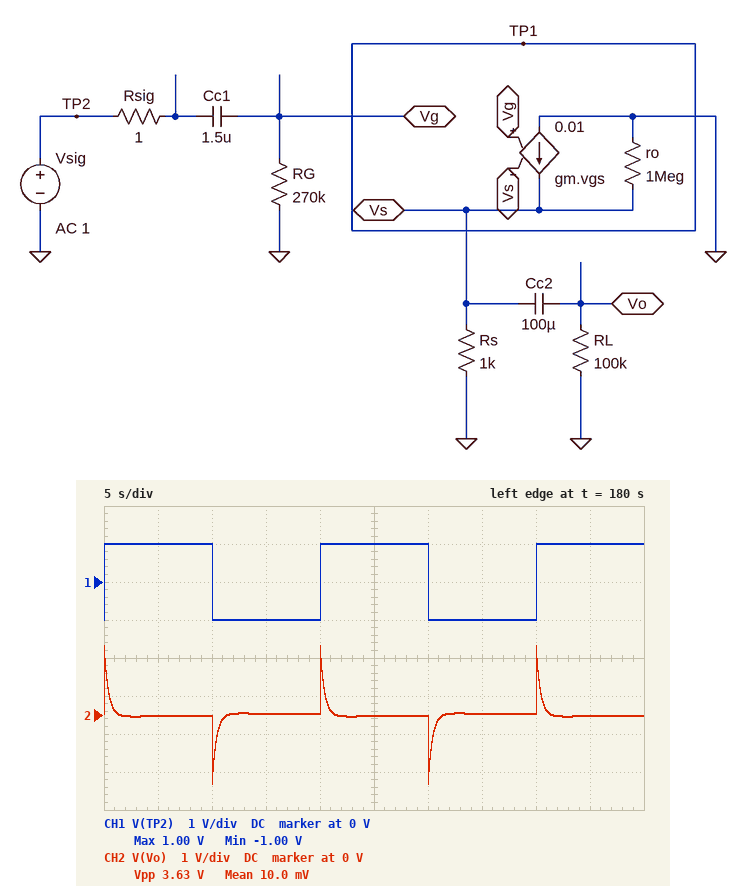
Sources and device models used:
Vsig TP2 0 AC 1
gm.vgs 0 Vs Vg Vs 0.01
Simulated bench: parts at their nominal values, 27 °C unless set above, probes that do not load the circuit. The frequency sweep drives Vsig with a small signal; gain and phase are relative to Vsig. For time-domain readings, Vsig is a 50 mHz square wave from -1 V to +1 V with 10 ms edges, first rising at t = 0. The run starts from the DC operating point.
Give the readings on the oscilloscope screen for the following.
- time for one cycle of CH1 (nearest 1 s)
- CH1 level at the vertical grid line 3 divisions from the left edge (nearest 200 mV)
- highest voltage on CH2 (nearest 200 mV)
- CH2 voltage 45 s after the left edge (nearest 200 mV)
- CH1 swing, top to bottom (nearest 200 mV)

20 s
-1.0 V
1.8 V
0 V
2.0 V
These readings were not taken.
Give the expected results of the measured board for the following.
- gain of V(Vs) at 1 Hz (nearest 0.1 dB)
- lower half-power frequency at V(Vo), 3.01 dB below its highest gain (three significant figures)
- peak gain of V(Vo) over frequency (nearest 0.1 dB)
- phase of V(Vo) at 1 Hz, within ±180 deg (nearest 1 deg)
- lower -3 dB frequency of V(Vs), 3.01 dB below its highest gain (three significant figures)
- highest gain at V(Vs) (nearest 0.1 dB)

-1.5 dB
394 mHz
-0.8 dB
22 deg
393 mHz
-0.8 dB
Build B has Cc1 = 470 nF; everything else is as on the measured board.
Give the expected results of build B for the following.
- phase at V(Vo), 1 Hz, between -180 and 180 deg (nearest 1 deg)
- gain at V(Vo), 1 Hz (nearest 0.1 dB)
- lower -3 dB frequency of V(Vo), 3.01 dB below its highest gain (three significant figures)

52 deg
-4.9 dB
1.25 Hz
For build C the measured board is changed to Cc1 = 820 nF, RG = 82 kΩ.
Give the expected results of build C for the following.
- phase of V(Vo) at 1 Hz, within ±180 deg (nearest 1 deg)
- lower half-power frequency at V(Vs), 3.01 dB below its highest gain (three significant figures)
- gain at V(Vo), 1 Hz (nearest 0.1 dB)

68 deg
2.37 Hz
-9.0 dB
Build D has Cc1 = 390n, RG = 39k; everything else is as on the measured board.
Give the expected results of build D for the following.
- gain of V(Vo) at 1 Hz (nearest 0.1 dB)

-21.3 dB
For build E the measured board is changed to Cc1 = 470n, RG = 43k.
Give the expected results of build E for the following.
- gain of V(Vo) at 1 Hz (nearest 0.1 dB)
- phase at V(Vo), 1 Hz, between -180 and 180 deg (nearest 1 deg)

-18.8 dB
84 deg
